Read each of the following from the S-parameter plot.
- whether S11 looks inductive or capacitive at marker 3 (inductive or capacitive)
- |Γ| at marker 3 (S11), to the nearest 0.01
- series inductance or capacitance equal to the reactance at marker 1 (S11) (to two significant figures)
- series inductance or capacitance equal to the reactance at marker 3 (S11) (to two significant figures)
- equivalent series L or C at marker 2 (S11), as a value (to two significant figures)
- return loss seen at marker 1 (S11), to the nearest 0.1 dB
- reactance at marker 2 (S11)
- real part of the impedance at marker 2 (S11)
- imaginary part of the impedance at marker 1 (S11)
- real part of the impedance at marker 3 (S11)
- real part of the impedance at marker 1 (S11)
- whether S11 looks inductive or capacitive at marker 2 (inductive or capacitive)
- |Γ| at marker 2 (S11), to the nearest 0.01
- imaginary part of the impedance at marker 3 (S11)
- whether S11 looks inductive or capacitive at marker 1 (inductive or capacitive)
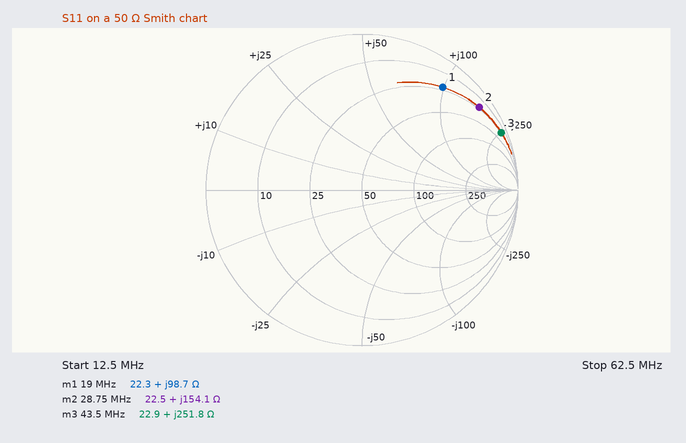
inductive
0.97
830 nH
920 nH
850 nH
1.5 dB
+154.1 Ω
22.5 Ω
+98.7 Ω
22.9 Ω
22.3 Ω
inductive
0.92
+251.8 Ω
inductive
